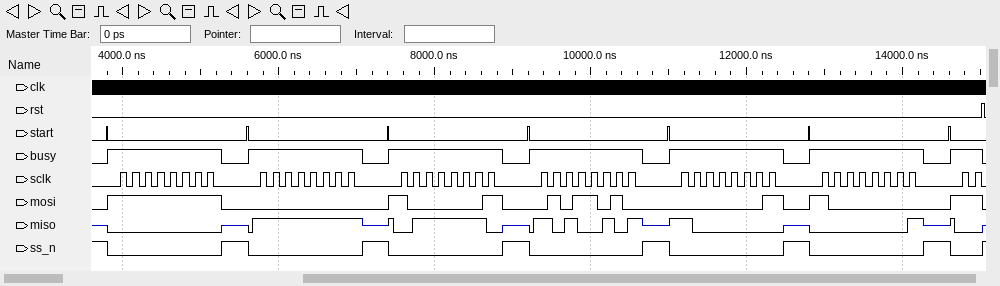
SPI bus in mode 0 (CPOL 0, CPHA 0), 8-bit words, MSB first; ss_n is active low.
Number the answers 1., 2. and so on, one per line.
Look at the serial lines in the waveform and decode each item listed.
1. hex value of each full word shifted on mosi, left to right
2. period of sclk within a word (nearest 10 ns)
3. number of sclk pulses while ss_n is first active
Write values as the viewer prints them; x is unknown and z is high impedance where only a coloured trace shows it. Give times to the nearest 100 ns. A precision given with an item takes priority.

1. FF, 00, 81, 5A, 01, 80
2. 160 ns
3. 8
